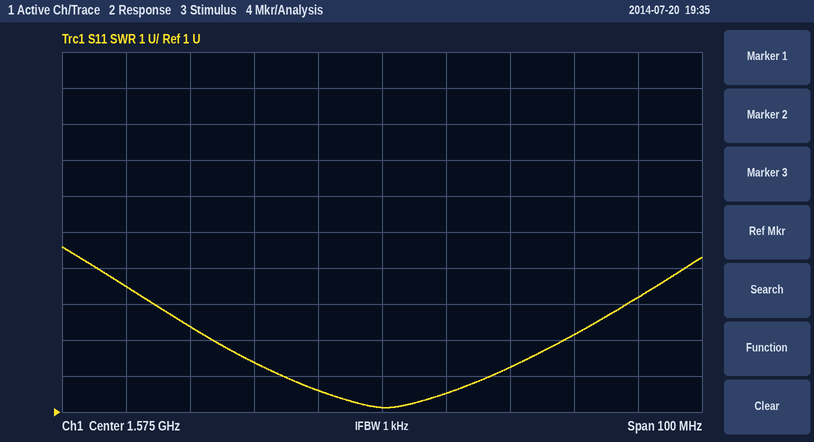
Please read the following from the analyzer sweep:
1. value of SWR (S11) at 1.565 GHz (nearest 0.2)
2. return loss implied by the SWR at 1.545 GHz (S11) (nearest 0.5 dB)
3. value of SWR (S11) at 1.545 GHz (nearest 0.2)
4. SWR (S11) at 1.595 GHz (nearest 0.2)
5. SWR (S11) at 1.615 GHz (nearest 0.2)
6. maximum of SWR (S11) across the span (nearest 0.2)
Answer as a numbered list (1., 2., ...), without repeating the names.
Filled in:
1. 1.6
2. 5.5 dB
3. 3.4
4. 2.2
5. 4.2
6. 5.6
